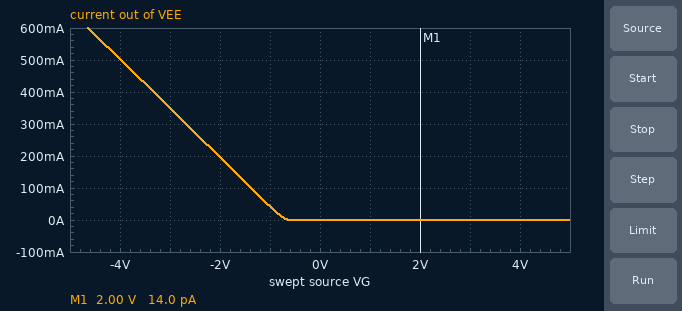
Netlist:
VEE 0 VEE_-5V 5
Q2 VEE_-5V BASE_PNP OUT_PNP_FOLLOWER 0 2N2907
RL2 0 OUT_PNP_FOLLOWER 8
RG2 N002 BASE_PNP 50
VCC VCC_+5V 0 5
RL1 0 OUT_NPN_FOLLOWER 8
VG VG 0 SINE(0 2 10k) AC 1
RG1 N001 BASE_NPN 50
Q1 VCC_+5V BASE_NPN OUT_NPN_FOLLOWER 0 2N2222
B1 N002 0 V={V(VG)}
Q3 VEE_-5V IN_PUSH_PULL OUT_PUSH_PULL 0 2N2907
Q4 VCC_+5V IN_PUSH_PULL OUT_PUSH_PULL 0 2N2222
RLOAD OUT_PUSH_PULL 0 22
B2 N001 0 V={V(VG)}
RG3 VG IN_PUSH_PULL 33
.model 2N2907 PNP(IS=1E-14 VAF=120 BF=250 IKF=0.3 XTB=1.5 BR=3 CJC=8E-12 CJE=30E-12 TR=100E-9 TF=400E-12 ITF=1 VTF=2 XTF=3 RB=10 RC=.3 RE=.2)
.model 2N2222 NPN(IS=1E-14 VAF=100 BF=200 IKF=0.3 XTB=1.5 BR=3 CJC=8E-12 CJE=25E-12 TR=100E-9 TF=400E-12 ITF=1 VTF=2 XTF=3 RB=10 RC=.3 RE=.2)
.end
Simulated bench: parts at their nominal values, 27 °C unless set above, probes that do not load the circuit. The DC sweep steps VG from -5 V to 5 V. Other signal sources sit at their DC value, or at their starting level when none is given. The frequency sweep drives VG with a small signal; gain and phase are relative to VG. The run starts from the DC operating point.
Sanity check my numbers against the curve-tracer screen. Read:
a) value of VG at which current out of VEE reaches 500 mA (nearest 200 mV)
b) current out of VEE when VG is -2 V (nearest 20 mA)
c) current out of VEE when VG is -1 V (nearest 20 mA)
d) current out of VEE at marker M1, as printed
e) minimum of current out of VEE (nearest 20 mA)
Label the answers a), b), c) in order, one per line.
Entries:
a) -4.0 V
b) 200 mA
c) 40 mA
d) 14.0 pA
e) 0 A
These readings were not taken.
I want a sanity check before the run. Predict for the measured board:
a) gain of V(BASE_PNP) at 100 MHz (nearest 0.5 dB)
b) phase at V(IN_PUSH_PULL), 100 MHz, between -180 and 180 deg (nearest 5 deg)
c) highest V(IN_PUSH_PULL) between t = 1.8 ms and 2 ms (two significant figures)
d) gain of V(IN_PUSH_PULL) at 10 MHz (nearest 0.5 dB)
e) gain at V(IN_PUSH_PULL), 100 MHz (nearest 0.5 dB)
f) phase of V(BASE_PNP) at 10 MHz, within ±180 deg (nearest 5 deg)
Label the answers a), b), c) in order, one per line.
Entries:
a) -4.5 dB
b) -25 deg
c) 2.0 V
d) 0 dB
e) -5.0 dB
f) -5 deg
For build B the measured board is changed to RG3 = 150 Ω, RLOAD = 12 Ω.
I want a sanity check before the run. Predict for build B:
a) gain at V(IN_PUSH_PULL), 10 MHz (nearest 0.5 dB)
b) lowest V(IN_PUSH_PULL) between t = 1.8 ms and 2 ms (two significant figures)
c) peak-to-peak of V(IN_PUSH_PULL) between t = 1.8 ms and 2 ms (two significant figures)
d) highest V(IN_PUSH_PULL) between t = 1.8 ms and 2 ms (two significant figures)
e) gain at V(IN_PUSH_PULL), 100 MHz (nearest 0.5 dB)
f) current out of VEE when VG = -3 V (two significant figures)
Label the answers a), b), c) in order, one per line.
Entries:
a) -1.5 dB
b) -1.9 V
c) 3.8 V
d) 1.9 V
e) -15.0 dB
f) 420 mA
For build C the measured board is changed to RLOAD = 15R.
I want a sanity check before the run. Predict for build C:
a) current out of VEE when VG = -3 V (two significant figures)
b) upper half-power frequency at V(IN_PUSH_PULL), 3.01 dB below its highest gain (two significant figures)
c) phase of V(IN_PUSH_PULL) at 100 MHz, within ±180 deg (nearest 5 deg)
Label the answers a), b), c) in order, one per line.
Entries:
a) 390 mA
b) 58 MHz
c) -30 deg
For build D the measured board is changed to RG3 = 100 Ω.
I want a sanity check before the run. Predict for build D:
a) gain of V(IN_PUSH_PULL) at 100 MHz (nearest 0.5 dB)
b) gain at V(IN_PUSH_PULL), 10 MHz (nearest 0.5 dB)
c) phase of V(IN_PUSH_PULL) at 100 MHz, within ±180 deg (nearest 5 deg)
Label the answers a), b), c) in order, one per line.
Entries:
a) -11.0 dB
b) -1.0 dB
c) -40 deg
